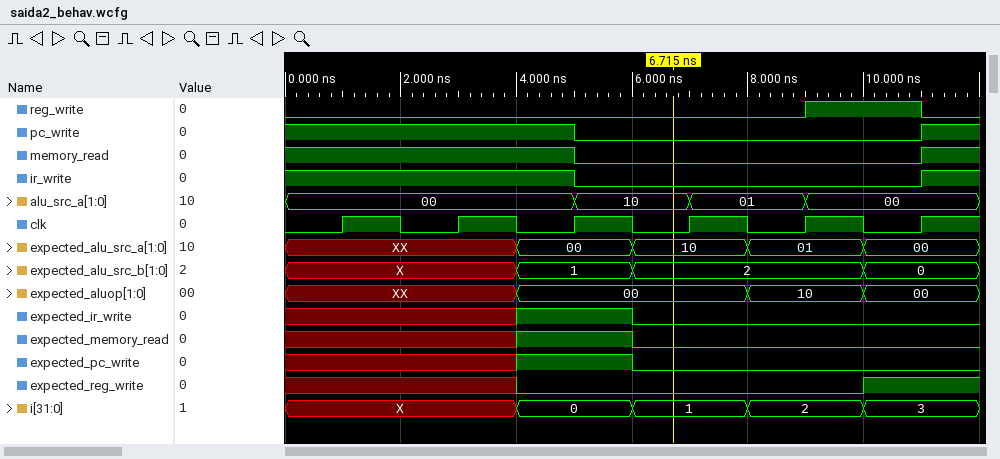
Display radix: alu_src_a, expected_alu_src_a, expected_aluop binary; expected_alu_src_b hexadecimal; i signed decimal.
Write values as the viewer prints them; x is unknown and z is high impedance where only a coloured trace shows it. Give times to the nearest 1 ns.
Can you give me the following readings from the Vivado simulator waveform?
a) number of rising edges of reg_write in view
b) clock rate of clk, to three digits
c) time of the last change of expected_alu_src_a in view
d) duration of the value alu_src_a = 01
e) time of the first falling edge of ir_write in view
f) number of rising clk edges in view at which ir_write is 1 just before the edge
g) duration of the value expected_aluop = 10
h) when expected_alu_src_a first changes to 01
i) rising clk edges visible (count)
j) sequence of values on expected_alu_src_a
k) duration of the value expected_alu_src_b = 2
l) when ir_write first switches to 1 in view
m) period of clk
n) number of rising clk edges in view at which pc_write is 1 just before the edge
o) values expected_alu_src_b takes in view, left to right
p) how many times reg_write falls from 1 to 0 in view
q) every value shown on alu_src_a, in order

1
500 MHz
10 ns
2 ns
5 ns
3
2 ns
8 ns
6
XX, 00, 10, 01, 00
4 ns
11 ns
2 ns
3
X, 1, 2, 0
1
00, 10, 01, 00
